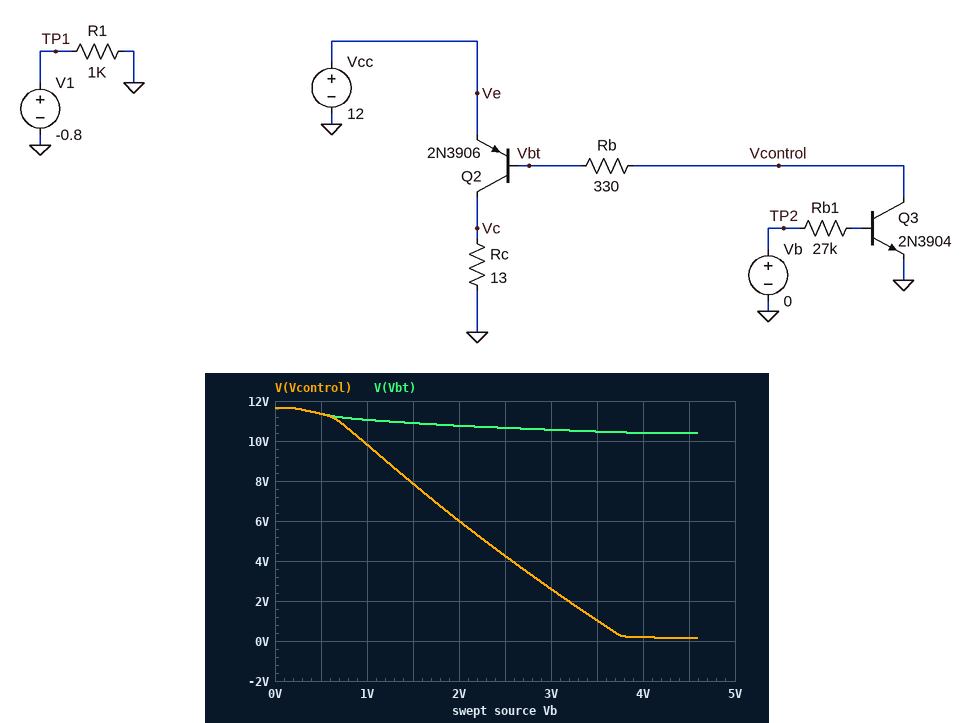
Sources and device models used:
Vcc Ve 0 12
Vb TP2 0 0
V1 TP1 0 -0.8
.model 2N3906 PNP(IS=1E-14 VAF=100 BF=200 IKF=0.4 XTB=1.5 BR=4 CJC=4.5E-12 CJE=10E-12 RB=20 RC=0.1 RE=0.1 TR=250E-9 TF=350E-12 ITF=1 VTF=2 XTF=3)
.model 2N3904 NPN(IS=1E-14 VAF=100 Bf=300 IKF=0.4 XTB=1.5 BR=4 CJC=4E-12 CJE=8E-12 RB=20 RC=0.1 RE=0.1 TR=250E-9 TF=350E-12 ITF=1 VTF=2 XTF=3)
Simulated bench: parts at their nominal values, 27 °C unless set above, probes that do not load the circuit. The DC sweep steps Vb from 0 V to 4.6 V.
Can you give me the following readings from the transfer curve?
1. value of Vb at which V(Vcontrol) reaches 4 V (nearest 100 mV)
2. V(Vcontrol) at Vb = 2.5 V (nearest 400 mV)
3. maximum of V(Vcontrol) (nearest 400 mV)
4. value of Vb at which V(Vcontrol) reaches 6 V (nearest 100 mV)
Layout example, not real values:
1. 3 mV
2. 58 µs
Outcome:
1. 2.6 V
2. 4.4 V
3. 11.6 V
4. 2.0 V
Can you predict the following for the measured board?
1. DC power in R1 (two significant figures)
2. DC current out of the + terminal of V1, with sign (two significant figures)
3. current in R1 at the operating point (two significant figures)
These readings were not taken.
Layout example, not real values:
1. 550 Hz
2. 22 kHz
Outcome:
1. 640 µW
2. -800 µA
3. 800 µA
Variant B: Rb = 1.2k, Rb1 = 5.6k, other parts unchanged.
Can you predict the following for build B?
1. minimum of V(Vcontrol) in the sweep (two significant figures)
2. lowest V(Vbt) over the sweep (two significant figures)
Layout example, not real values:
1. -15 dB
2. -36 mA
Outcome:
1. 43 mV
2. 11 V
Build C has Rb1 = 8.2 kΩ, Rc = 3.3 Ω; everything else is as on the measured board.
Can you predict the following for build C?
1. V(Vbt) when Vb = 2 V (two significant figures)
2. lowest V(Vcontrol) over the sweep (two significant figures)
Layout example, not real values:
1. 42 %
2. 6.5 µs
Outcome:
1. 10 V
2. 90 mV
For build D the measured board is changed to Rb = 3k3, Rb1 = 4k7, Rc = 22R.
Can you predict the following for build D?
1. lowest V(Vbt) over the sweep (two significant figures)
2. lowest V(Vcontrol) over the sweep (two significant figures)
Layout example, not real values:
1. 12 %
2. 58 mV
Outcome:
1. 11 V
2. 23 mV
